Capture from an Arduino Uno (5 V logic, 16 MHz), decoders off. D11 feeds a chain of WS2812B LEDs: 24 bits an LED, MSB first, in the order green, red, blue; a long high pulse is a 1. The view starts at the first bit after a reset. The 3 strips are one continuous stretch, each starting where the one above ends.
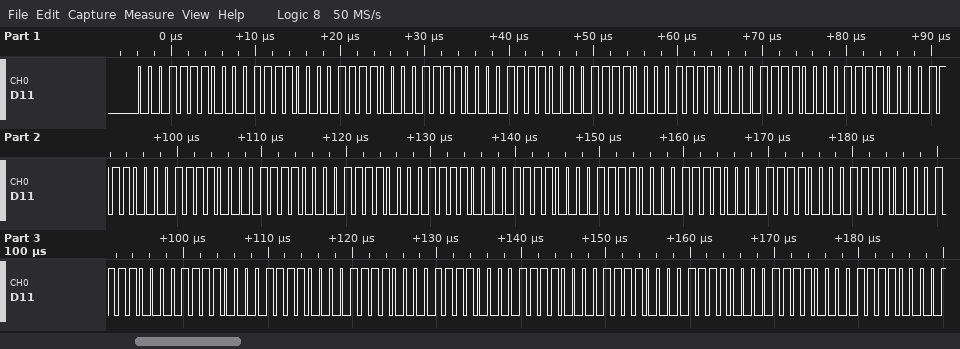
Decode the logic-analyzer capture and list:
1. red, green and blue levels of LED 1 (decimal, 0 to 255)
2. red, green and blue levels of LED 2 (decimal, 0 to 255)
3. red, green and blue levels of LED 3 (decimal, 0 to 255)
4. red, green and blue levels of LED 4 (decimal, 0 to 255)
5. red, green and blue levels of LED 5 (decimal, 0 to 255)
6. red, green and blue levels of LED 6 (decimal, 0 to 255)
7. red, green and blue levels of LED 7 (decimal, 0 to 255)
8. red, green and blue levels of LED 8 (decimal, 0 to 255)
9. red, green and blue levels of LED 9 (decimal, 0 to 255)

30, 30, 30
30, 30, 30
30, 30, 30
30, 30, 30
30, 30, 30
30, 30, 30
30, 30, 30
30, 30, 30
30, 30, 30
